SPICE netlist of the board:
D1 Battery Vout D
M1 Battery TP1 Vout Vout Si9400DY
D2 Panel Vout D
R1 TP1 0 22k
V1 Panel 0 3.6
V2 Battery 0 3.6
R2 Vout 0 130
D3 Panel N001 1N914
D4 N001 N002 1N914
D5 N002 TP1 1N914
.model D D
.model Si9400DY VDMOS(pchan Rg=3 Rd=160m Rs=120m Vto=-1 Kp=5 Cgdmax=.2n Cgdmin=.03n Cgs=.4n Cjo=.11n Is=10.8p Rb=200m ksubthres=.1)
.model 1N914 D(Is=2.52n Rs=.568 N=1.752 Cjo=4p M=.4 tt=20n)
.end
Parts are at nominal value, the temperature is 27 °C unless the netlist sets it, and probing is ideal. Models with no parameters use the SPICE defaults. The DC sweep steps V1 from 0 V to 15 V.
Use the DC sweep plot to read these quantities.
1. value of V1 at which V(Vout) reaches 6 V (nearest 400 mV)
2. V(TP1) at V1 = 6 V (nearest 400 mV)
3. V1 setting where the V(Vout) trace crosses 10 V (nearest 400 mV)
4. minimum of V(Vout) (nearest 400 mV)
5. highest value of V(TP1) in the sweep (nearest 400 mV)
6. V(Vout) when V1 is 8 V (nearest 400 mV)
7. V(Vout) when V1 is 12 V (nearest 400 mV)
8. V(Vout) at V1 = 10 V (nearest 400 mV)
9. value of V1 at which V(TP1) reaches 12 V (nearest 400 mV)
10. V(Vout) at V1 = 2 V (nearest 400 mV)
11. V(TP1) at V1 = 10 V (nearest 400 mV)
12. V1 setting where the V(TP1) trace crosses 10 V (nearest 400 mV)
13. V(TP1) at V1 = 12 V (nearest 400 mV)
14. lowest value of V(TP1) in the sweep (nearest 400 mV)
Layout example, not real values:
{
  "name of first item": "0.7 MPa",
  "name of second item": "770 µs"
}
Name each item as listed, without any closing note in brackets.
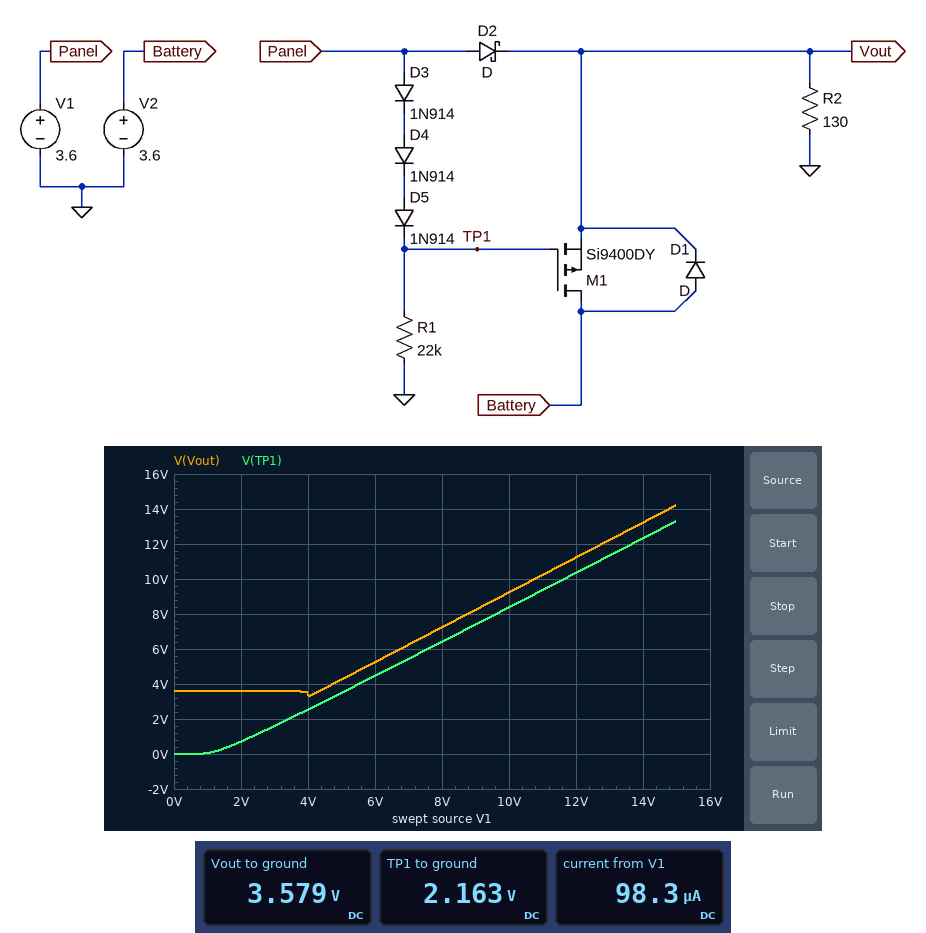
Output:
{
  "value of V1 at which V(Vout) reaches 6 V": "6.8 V",
  "V(TP1) at V1 = 6 V": "4.4 V",
  "V1 setting where the V(Vout) trace crosses 10 V": "10.8 V",
  "minimum of V(Vout)": "3.2 V",
  "highest value of V(TP1) in the sweep": "13.2 V",
  "V(Vout) when V1 is 8 V": "7.2 V",
  "V(Vout) when V1 is 12 V": "11.2 V",
  "V(Vout) at V1 = 10 V": "9.2 V",
  "value of V1 at which V(TP1) reaches 12 V": "13.6 V",
  "V(Vout) at V1 = 2 V": "3.6 V",
  "V(TP1) at V1 = 10 V": "8.4 V",
  "V1 setting where the V(TP1) trace crosses 10 V": "11.6 V",
  "V(TP1) at V1 = 12 V": "10.4 V",
  "lowest value of V(TP1) in the sweep": "0 V"
}
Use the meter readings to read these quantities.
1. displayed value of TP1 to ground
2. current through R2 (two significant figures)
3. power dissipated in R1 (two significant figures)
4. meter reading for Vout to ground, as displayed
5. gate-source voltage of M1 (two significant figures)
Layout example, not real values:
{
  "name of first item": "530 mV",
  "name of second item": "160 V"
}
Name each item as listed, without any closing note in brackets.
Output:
{
  "displayed value of TP1 to ground": "2.163 V",
  "current through R2": "28 mA",
  "power dissipated in R1": "210 µW",
  "meter reading for Vout to ground, as displayed": "3.579 V",
  "gate-source voltage of M1": "-1.4 V"
}
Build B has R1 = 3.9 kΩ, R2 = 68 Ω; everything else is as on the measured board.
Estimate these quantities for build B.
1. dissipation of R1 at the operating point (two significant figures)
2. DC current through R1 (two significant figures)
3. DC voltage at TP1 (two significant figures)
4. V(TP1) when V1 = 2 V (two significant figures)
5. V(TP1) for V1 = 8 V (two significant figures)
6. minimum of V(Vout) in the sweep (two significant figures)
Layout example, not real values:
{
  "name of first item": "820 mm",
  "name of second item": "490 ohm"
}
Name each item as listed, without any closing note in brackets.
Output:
{
  "dissipation of R1 at the operating point": "970 µW",
  "DC current through R1": "500 µA",
  "DC voltage at TP1": "1.9 V",
  "V(TP1) when V1 = 2 V": "520 mV",
  "V(TP1) for V1 = 8 V": "6.2 V",
  "minimum of V(Vout) in the sweep": "3.5 V"
}
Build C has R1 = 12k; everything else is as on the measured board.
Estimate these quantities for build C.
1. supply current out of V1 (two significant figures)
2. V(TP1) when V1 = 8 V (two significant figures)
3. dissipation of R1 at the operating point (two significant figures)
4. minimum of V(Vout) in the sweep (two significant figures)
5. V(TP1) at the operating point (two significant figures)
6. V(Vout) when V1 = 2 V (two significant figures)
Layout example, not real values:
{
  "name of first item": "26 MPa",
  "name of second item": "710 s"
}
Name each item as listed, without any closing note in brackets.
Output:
{
  "supply current out of V1": "170 µA",
  "V(TP1) when V1 = 8 V": "6.3 V",
  "dissipation of R1 at the operating point": "360 µW",
  "minimum of V(Vout) in the sweep": "3.4 V",
  "V(TP1) at the operating point": "2.1 V",
  "V(Vout) when V1 = 2 V": "3.6 V"
}
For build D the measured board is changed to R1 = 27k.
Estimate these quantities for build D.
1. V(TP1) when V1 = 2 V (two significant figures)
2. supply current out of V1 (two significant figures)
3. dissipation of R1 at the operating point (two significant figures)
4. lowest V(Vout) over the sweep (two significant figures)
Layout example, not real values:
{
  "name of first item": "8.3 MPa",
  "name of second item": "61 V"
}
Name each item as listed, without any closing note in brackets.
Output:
{
  "V(TP1) when V1 = 2 V": "740 mV",
  "supply current out of V1": "81 µA",
  "dissipation of R1 at the operating point": "180 µW",
  "lowest V(Vout) over the sweep": "3.3 V"
}
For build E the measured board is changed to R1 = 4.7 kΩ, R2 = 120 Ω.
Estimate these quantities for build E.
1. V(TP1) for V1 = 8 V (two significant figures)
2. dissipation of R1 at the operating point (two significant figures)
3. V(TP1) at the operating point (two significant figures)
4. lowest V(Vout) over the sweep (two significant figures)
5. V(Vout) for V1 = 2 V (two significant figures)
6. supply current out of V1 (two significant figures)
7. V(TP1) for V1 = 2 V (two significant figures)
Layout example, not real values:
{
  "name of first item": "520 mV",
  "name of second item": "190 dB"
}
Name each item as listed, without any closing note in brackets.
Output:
{
  "V(TP1) for V1 = 8 V": "6.2 V",
  "dissipation of R1 at the operating point": "820 µW",
  "V(TP1) at the operating point": "2.0 V",
  "lowest V(Vout) over the sweep": "3.5 V",
  "V(Vout) for V1 = 2 V": "3.6 V",
  "supply current out of V1": "420 µA",
  "V(TP1) for V1 = 2 V": "540 mV"
}
